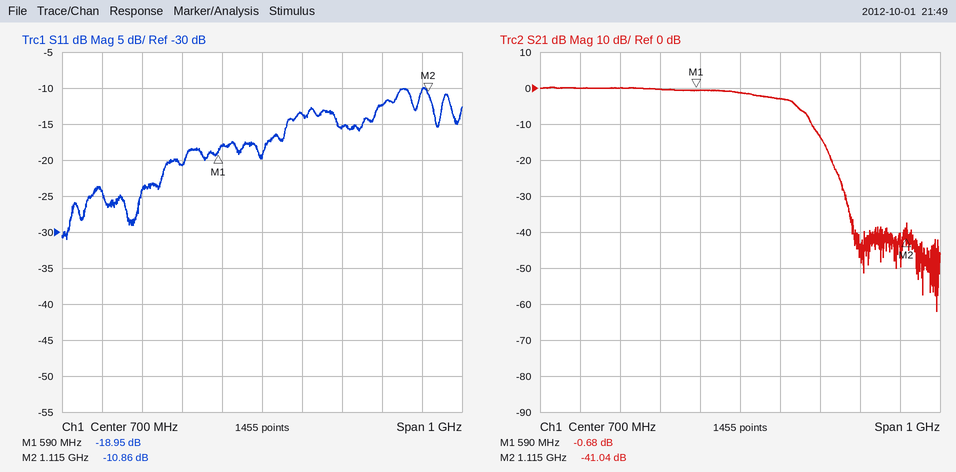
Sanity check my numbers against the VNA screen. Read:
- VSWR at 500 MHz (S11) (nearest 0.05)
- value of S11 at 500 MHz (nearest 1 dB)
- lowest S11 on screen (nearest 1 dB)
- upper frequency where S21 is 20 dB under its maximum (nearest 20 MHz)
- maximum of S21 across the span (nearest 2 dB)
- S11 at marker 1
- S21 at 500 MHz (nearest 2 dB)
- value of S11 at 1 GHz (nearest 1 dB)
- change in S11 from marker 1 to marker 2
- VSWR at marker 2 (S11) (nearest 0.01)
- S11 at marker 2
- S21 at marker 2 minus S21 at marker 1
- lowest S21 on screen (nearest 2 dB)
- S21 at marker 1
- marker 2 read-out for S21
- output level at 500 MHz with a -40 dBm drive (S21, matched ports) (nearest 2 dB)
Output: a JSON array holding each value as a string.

["1.20", "-21 dB", "-31 dB", "920 MHz", "0 dB", "-18.95 dB", "0 dB", "-12 dB", "8.09 dB", "1.80", "-10.86 dB", "-40.36 dB", "-62 dB", "-0.68 dB", "-41.04 dB", "-40 dBm"]
